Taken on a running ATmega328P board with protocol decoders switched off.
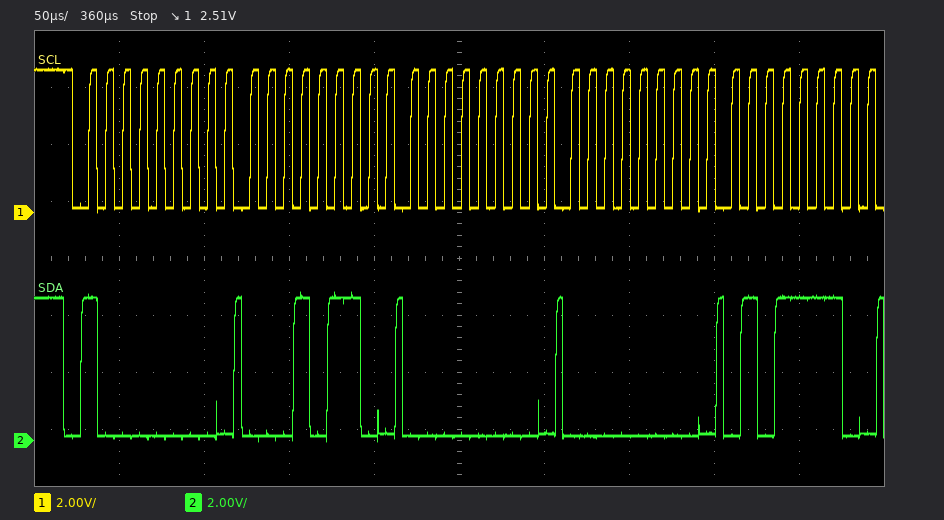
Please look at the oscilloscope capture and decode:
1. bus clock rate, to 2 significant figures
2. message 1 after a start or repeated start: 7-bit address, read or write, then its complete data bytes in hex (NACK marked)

100 kHz
0x40 write: 16 00 00 5E
